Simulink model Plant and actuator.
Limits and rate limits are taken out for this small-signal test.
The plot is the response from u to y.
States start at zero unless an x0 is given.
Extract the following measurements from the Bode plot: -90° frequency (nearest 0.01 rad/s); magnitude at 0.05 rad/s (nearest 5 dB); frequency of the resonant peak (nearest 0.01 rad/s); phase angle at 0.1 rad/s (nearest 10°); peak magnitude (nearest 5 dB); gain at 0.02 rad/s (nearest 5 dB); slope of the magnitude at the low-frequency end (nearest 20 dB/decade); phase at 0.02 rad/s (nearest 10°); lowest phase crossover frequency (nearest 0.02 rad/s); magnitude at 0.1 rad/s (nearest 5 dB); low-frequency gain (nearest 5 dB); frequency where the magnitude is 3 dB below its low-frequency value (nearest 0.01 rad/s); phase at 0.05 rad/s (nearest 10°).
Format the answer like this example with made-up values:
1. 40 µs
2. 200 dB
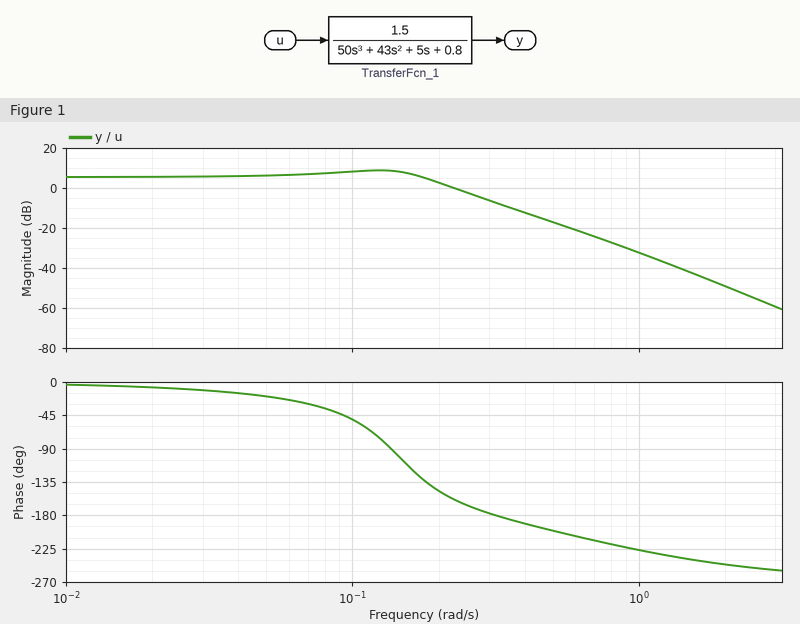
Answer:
1. 0.14 rad/s
2. 5 dB
3. 0.12 rad/s
4. -50°
5. 10 dB
6. 5 dB
7. 0 dB/decade
8. -10°
9. 0.32 rad/s
10. 10 dB
11. 5 dB
12. 0.20 rad/s
13. -20°
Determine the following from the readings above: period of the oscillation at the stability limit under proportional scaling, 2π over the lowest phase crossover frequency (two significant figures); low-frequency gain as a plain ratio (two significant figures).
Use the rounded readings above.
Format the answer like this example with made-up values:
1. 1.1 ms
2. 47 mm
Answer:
1. 20 s
2. 1.8
